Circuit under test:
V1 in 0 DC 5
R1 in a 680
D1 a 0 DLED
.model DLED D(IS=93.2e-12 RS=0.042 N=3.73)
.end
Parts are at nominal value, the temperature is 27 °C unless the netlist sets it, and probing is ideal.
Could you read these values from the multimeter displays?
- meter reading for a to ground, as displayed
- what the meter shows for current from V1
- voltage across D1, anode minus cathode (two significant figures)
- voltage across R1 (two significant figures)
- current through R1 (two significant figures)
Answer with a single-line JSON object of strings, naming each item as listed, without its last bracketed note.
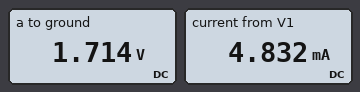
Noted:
{"meter reading for a to ground, as displayed": "1.714 V", "what the meter shows for current from V1": "4.832 mA", "voltage across D1, anode minus cathode": "1.7 V", "voltage across R1": "3.3 V", "current through R1": "4.8 mA"}
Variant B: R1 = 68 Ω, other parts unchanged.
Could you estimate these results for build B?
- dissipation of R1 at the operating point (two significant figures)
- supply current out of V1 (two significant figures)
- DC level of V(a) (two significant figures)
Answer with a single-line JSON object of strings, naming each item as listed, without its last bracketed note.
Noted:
{"dissipation of R1 at the operating point": "140 mW", "supply current out of V1": "45 mA", "DC level of V(a)": "1.9 V"}
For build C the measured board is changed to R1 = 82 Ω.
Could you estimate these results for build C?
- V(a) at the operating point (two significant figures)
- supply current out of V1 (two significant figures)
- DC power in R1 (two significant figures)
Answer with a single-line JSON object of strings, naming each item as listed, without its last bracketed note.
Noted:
{"V(a) at the operating point": "1.9 V", "supply current out of V1": "38 mA", "DC power in R1": "120 mW"}
